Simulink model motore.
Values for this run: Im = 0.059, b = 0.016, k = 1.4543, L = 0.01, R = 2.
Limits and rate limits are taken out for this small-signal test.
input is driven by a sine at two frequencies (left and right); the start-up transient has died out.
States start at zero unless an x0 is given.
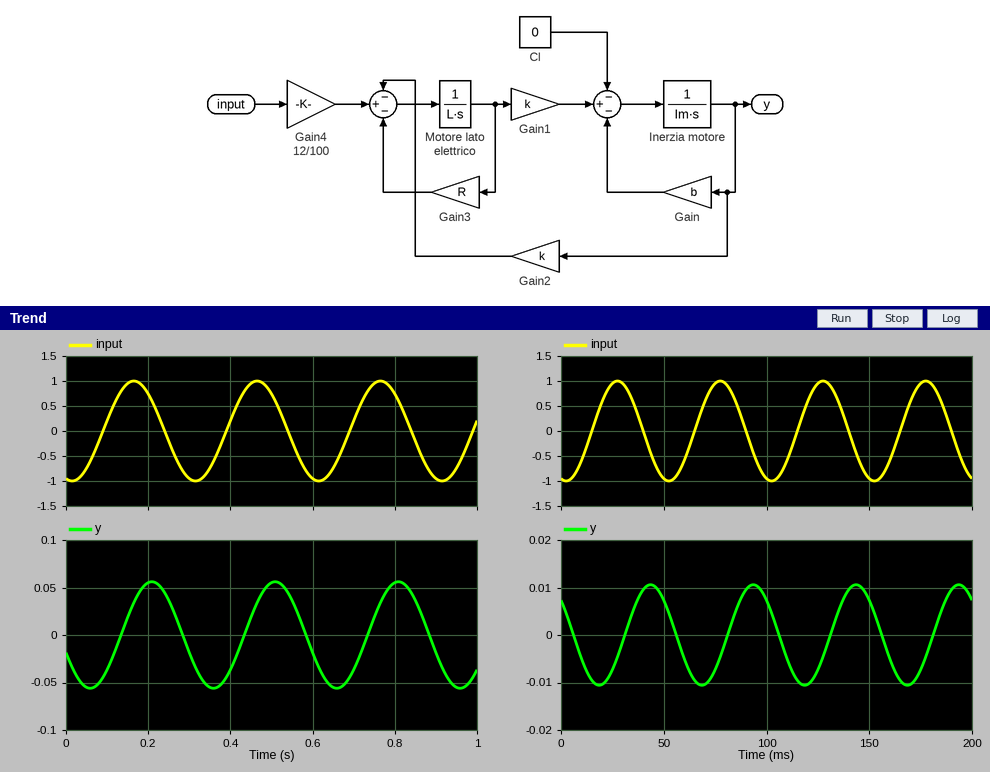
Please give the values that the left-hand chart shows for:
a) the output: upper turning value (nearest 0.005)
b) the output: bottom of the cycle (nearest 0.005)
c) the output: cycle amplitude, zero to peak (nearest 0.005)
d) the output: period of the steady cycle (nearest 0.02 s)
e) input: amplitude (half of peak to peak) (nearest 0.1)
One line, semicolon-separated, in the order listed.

0.055; -0.055; 0.055; 0.30 s; 1.0
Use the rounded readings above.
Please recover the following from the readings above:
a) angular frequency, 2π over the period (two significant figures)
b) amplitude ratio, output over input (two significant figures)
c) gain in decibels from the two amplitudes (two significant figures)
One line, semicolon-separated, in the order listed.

21 rad/s; 0.055; -25 dB
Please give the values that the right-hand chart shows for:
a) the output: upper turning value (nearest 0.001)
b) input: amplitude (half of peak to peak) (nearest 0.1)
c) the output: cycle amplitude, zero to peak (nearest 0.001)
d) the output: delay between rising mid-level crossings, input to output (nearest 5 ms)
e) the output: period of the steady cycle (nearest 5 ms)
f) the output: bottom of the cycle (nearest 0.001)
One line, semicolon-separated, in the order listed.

0.011; 1.0; 0.011; 15 ms; 50 ms; -0.011
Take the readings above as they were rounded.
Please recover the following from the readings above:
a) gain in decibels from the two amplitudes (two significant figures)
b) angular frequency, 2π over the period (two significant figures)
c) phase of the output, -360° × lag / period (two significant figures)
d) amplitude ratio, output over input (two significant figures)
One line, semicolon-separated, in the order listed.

-39 dB; 0.13 rad/ms; -110°; 0.011
